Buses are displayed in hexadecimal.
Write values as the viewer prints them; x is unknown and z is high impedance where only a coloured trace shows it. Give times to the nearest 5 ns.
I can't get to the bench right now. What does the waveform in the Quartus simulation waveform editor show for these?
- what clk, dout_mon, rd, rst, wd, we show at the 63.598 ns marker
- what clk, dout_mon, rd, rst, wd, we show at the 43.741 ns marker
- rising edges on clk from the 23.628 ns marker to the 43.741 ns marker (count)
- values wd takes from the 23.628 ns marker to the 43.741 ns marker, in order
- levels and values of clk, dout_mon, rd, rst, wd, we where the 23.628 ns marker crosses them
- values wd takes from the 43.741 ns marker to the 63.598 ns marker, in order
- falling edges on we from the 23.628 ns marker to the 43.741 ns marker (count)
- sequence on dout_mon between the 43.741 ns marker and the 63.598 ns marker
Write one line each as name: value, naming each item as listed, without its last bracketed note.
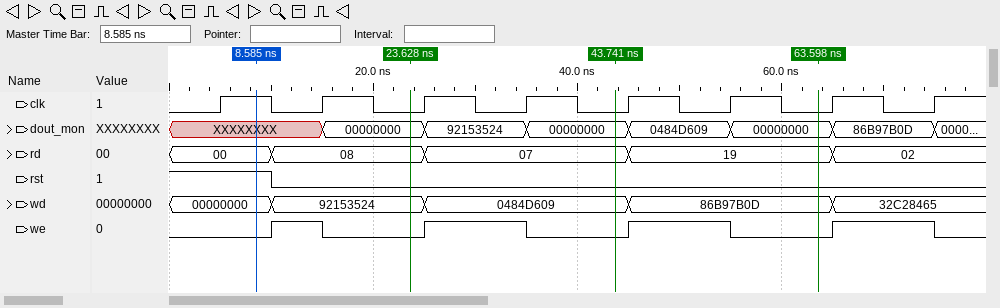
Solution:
what clk, dout_mon, rd, rst, wd, we show at the 63.598 ns marker: clk=0, dout_mon=00000000, rd=19, rst=0, wd=86B97B0D, we=0
what clk, dout_mon, rd, rst, wd, we show at the 43.741 ns marker: clk=0, dout_mon=00000000, rd=07, rst=0, wd=0484D609, we=0
rising edges on clk from the 23.628 ns marker to the 43.741 ns marker: 2
values wd takes from the 23.628 ns marker to the 43.741 ns marker, in order: 92153524, 0484D609
levels and values of clk, dout_mon, rd, rst, wd, we where the 23.628 ns marker crosses them: clk=0, dout_mon=00000000, rd=08, rst=0, wd=92153524, we=0
values wd takes from the 43.741 ns marker to the 63.598 ns marker, in order: 0484D609, 86B97B0D
falling edges on we from the 23.628 ns marker to the 43.741 ns marker: 1
sequence on dout_mon between the 43.741 ns marker and the 63.598 ns marker: 00000000, 0484D609, 00000000
